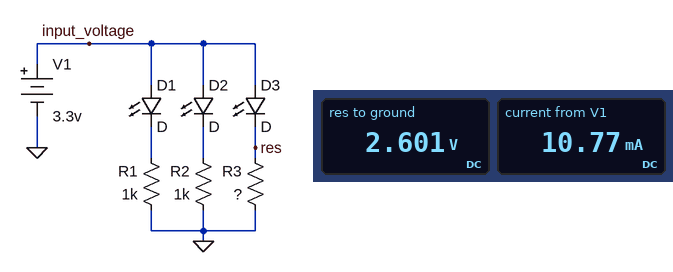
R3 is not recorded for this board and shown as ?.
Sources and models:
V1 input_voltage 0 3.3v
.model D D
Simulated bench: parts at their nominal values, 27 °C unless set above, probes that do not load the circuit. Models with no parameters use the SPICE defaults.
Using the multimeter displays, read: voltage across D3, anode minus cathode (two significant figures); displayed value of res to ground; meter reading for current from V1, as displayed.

700 mV
2.601 V
10.77 mA
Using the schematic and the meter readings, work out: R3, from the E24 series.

470 Ω
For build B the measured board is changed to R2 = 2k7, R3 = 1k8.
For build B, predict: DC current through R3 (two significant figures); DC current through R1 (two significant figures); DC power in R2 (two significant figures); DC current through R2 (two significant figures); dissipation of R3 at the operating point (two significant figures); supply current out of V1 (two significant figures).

1.5 mA
2.6 mA
2.6 mW
980 µA
3.9 mW
5.1 mA
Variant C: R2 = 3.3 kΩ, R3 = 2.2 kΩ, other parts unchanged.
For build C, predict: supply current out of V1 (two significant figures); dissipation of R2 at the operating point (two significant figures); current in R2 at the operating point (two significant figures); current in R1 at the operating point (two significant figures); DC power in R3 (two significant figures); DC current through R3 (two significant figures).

4.6 mA
2.1 mW
800 µA
2.6 mA
3.2 mW
1.2 mA
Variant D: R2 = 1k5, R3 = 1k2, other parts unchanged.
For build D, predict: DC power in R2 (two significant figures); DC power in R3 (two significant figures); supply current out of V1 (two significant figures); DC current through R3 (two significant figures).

4.6 mW
5.7 mW
6.6 mA
2.2 mA
